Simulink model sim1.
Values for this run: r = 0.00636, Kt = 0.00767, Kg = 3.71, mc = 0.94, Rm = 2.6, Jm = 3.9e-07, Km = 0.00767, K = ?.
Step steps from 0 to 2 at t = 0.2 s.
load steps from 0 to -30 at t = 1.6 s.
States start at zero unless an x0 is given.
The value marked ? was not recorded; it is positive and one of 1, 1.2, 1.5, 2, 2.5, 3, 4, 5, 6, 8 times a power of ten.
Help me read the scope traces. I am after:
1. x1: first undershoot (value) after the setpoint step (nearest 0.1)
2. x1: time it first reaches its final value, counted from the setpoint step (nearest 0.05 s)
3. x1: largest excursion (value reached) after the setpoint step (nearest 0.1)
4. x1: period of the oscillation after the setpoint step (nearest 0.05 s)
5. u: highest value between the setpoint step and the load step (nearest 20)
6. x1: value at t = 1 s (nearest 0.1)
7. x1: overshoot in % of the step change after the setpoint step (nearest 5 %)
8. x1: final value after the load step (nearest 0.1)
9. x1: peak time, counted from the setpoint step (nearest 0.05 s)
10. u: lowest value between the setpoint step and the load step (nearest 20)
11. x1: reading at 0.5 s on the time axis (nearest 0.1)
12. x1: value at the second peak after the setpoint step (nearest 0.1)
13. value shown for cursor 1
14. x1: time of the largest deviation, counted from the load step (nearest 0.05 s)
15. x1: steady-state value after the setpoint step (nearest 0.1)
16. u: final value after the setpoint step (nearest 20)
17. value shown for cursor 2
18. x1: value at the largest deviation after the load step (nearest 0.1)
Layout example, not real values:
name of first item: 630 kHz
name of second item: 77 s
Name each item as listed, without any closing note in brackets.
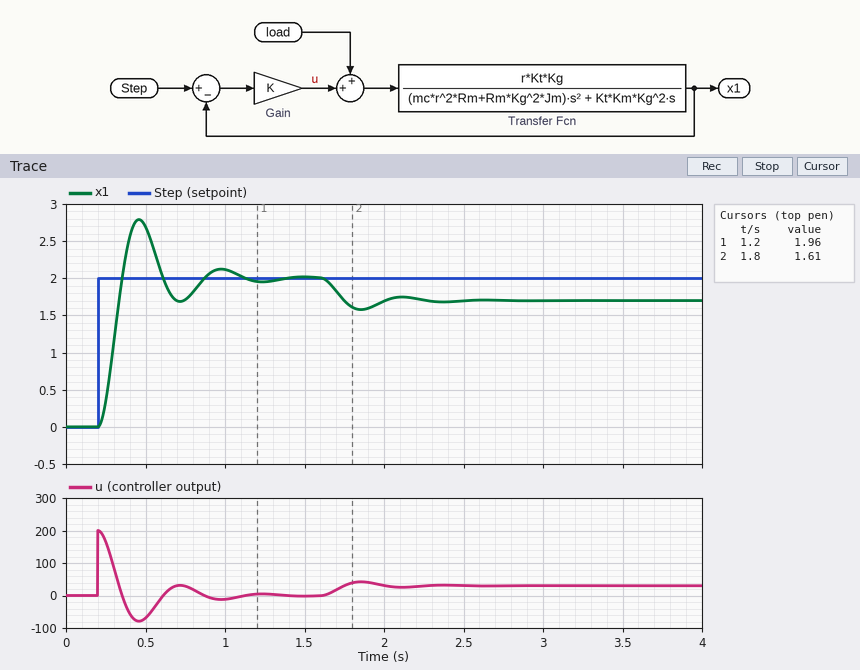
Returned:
x1: first undershoot (value) after the setpoint step: 1.7
x1: time it first reaches its final value, counted from the setpoint step: 0.15 s
x1: largest excursion (value reached) after the setpoint step: 2.8
x1: period of the oscillation after the setpoint step: 0.50 s
u: highest value between the setpoint step and the load step: 200
x1: value at t = 1 s: 2.1
x1: overshoot in % of the step change after the setpoint step: 40 %
x1: final value after the load step: 1.7
x1: peak time, counted from the setpoint step: 0.25 s
u: lowest value between the setpoint step and the load step: -80
x1: reading at 0.5 s on the time axis: 2.7
x1: value at the second peak after the setpoint step: 2.1
value shown for cursor 1: 1.96
x1: time of the largest deviation, counted from the load step: 0.25 s
x1: steady-state value after the setpoint step: 2.0
u: final value after the setpoint step: 0
value shown for cursor 2: 1.61
x1: value at the largest deviation after the load step: 1.6
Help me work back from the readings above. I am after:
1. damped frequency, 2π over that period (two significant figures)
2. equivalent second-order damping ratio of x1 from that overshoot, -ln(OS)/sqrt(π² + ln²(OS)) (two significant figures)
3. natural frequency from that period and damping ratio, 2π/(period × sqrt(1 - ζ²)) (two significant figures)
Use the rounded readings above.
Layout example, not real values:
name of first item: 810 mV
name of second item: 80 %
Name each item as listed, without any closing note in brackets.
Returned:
damped frequency, 2π over that period: 13 rad/s
equivalent second-order damping ratio of x1 from that overshoot, -ln(OS)/sqrt(π² + ln²(OS)): 0.28
natural frequency from that period and damping ratio, 2π/(period × sqrt(1 - ζ²)): 13 rad/s
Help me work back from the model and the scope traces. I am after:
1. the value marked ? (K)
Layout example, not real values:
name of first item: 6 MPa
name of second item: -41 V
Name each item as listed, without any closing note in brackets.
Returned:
the value marked ?: 100
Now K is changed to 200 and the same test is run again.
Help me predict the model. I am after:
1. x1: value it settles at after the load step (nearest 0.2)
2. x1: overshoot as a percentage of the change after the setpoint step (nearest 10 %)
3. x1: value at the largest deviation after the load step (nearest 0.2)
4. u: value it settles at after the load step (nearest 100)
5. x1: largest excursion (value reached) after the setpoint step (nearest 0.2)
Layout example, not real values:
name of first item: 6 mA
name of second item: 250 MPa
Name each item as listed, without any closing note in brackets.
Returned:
x1: value it settles at after the load step: 1.8
x1: overshoot as a percentage of the change after the setpoint step: 50 %
x1: value at the largest deviation after the load step: 1.8
u: value it settles at after the load step: 0
x1: largest excursion (value reached) after the setpoint step: 3.0
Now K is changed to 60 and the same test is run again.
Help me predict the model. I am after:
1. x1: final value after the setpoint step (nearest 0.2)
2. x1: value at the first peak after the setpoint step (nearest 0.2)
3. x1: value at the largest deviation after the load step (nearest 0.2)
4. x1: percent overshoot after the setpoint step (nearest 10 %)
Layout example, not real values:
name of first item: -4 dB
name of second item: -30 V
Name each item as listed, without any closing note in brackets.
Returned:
x1: final value after the setpoint step: 2.0
x1: value at the first peak after the setpoint step: 2.6
x1: value at the largest deviation after the load step: 1.4
x1: percent overshoot after the setpoint step: 30 %
